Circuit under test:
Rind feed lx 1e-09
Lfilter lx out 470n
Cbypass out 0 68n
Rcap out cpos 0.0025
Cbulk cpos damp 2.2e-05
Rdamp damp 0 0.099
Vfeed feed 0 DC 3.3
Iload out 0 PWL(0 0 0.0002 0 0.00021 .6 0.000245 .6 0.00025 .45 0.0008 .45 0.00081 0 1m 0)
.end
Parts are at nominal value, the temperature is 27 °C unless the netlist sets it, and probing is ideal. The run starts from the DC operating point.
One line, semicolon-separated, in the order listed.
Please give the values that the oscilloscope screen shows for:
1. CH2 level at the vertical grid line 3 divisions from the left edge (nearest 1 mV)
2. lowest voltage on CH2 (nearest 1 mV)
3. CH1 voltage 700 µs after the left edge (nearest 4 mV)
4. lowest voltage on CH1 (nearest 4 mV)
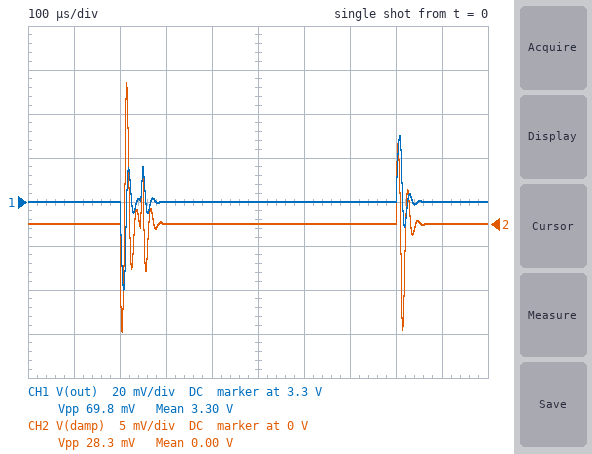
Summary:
0 V; -12 mV; 3.300 V; 3.260 V
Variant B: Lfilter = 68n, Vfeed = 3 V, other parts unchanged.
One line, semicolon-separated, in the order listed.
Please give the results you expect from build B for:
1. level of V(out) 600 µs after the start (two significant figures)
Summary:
3.0 V
